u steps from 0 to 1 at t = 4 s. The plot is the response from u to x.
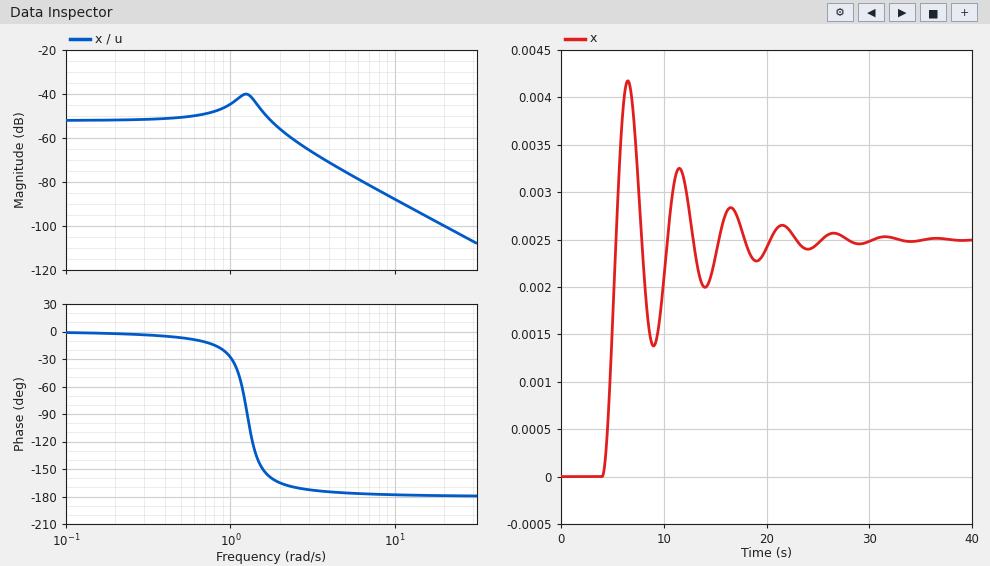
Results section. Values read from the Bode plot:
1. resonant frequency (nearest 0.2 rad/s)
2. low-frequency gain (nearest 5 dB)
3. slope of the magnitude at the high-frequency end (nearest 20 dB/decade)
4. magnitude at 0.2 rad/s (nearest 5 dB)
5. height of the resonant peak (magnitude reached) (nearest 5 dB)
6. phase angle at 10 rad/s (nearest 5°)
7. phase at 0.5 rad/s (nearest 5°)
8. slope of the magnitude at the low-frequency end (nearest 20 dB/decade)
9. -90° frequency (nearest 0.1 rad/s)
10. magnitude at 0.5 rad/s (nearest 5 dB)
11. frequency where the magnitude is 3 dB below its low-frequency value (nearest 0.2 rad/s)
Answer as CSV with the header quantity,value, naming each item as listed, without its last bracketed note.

quantity,value
resonant frequency,1.2 rad/s
low-frequency gain,-50 dB
slope of the magnitude at the high-frequency end,-40 dB/decade
magnitude at 0.2 rad/s,-50 dB
height of the resonant peak (magnitude reached),-40 dB
phase angle at 10 rad/s,-180°
phase at 0.5 rad/s,-5°
slope of the magnitude at the low-frequency end,0 dB/decade
-90° frequency,1.3 rad/s
magnitude at 0.5 rad/s,-50 dB
frequency where the magnitude is 3 dB below its low-frequency value,2.0 rad/s
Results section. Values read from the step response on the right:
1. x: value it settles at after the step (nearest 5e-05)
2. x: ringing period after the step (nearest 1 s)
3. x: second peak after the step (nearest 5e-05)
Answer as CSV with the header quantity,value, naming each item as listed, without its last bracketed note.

quantity,value
x: value it settles at after the step,0.00250
x: ringing period after the step,5 s
x: second peak after the step,0.00325
